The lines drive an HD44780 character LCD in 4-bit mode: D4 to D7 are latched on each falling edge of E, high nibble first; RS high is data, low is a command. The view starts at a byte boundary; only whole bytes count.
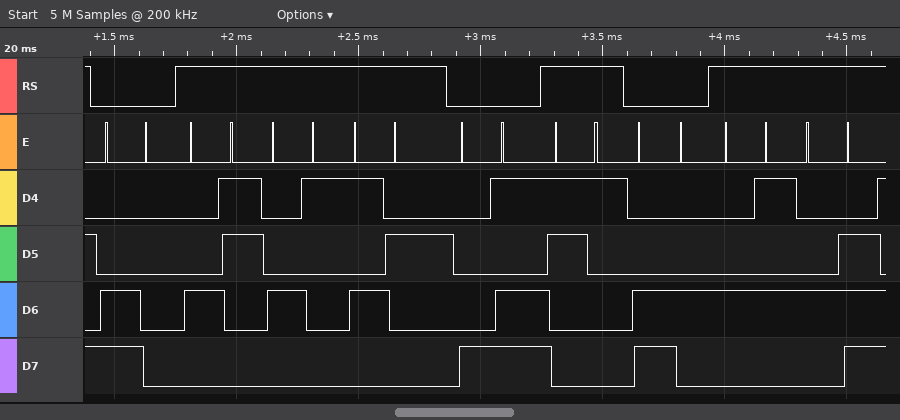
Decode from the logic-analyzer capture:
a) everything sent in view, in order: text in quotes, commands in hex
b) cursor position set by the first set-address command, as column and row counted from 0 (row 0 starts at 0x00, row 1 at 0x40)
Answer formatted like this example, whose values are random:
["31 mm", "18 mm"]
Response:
["0xC0 \"CAR\" 0x8D \"1\" 0xC4 \"EN\"", "column 0, row 1"]
